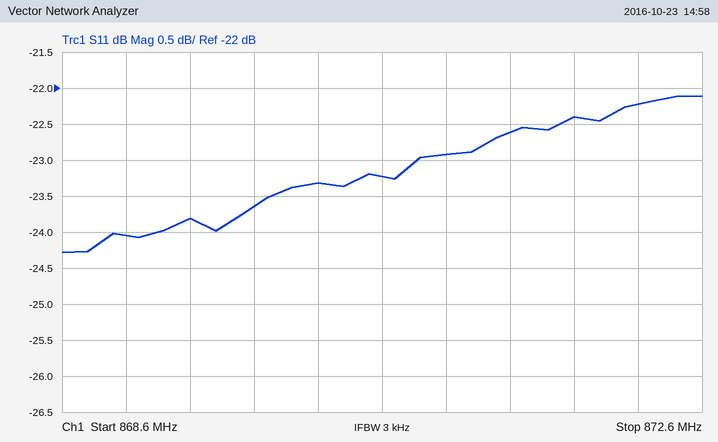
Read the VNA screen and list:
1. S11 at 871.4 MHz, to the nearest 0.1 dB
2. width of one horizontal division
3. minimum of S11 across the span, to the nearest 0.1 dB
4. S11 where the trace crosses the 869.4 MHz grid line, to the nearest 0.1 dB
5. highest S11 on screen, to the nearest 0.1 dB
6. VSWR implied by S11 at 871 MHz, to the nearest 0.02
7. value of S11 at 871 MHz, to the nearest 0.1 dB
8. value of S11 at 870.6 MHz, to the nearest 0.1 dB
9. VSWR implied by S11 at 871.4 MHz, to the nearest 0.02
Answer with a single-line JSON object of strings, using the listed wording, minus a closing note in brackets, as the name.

{"S11 at 871.4 MHz, to the nearest 0.1 dB": "-22.6 dB", "width of one horizontal division": "400 kHz", "minimum of S11 across the span, to the nearest 0.1 dB": "-24.3 dB", "S11 where the trace crosses the 869.4 MHz grid line, to the nearest 0.1 dB": "-23.8 dB", "highest S11 on screen, to the nearest 0.1 dB": "-22.1 dB", "VSWR implied by S11 at 871 MHz, to the nearest 0.02": "1.16", "value of S11 at 871 MHz, to the nearest 0.1 dB": "-22.9 dB", "value of S11 at 870.6 MHz, to the nearest 0.1 dB": "-23.2 dB", "VSWR implied by S11 at 871.4 MHz, to the nearest 0.02": "1.16"}
